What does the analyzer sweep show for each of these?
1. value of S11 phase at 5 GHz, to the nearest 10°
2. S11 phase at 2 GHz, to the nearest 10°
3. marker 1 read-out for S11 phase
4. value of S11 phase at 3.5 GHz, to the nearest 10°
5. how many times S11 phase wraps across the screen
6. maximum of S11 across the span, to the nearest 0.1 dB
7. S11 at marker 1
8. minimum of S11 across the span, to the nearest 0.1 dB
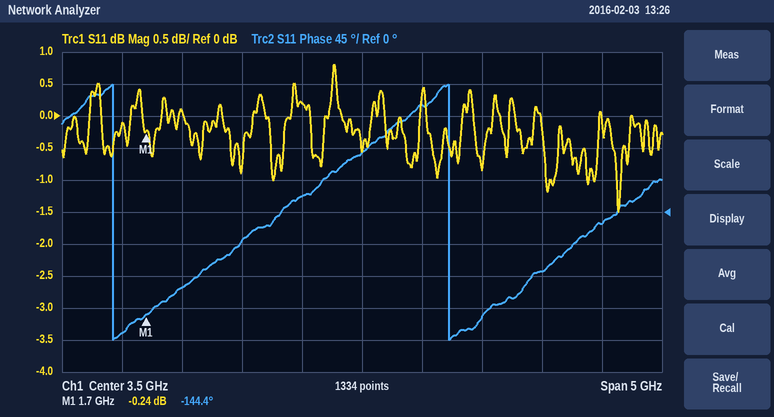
-80°
-110°
-144.4°
80°
2
0.8 dB
-0.24 dB
-1.5 dB
